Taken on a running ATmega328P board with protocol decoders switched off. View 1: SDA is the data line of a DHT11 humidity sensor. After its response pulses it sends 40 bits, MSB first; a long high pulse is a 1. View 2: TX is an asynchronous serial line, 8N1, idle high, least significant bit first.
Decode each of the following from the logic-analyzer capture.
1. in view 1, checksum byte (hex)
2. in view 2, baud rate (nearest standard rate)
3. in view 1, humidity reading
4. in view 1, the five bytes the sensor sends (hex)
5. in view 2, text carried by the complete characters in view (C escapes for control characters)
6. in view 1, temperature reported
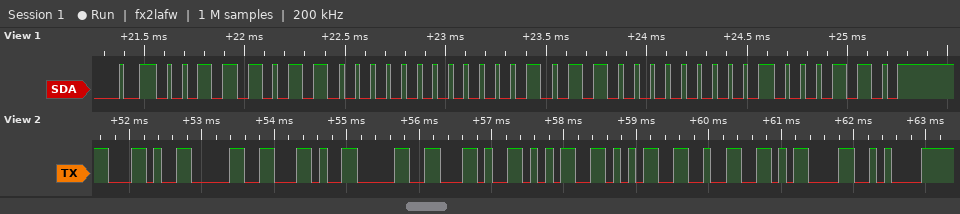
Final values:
0x46
9600 baud
59 %
3B 00 0B 00 46
",0,0,552\r\n"
11.0 °C
